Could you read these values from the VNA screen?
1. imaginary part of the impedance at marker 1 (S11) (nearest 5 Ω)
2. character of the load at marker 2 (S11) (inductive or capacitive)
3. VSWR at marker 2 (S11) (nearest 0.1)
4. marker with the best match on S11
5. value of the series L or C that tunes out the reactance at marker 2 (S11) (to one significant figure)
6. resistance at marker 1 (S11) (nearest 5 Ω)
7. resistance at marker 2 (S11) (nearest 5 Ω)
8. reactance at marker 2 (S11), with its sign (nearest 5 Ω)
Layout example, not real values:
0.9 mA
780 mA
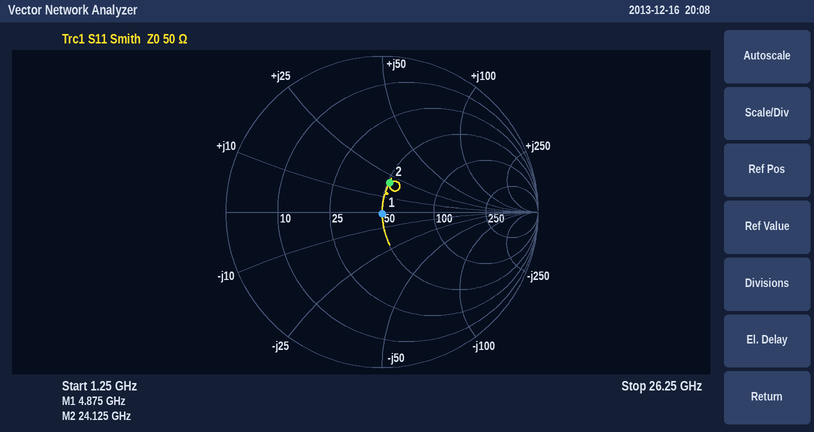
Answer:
0 Ω
inductive
1.5
marker 1
300 fF
50 Ω
50 Ω
+20 Ω
